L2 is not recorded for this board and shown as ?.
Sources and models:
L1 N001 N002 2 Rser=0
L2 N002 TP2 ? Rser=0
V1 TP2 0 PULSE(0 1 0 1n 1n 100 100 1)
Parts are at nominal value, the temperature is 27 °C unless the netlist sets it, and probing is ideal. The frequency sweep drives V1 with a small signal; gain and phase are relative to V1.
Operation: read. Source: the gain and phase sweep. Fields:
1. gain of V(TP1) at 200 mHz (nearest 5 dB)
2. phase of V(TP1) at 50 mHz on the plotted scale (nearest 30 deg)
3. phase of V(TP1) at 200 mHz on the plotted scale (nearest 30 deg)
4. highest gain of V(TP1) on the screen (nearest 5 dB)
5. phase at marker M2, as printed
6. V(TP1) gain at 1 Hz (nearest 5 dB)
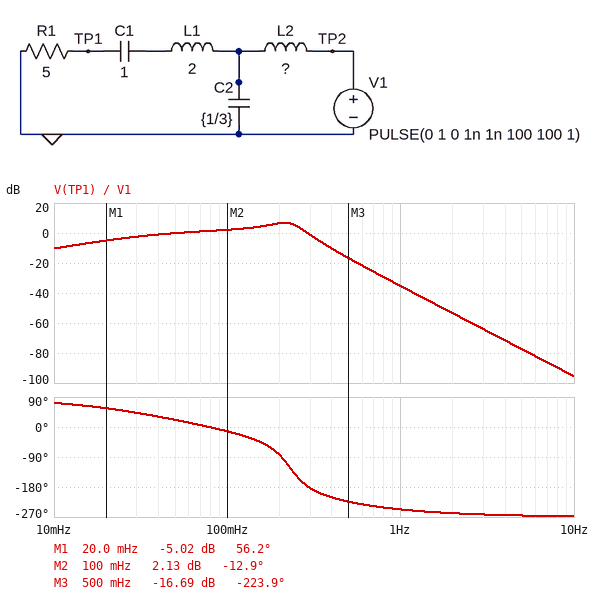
5 dB
30 deg
-90 deg
5 dB
-12.9 deg
-35 dB
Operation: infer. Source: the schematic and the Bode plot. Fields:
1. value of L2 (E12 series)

1.8 H
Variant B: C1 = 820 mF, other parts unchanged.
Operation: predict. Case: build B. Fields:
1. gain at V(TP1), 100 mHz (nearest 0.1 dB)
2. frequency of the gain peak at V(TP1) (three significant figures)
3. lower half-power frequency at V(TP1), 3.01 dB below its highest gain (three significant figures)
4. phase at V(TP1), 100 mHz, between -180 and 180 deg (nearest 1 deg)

2.2 dB
212 mHz
137 mHz
-9 deg
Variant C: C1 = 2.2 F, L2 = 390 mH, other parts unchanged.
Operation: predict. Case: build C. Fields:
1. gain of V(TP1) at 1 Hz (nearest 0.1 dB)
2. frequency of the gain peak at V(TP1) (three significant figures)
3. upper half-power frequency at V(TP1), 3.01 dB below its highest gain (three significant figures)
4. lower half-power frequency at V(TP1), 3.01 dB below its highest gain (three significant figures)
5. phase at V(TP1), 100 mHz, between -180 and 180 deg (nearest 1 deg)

-20.6 dB
465 mHz
486 mHz
442 mHz
-9 deg
